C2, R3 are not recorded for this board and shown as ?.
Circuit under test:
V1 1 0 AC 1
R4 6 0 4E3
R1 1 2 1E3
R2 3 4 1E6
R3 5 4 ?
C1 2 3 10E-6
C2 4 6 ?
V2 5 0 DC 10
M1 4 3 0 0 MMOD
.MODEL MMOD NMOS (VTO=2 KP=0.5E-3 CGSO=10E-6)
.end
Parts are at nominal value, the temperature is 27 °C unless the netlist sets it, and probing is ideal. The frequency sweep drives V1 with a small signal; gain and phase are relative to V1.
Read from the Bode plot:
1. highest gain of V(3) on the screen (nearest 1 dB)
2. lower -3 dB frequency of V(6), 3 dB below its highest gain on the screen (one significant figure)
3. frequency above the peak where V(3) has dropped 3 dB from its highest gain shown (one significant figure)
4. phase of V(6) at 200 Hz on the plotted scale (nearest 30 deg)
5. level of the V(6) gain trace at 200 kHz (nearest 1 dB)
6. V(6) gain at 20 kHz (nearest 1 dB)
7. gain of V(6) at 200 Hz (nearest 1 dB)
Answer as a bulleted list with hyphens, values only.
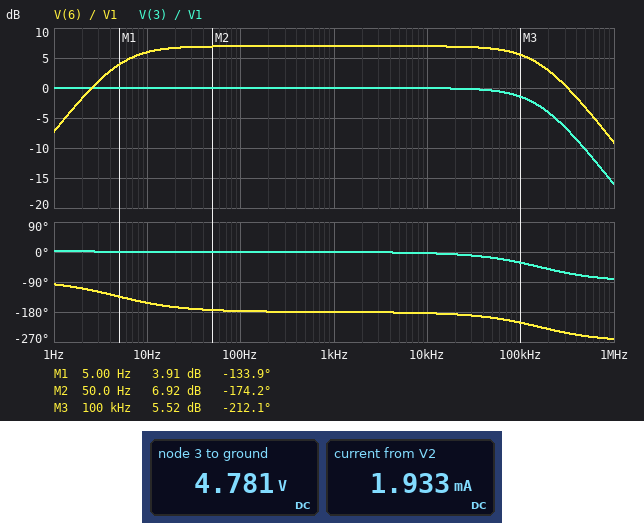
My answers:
- 0 dB
- 5 Hz
- 200 kHz
- -180 deg
- 3 dB
- 7 dB
- 7 dB
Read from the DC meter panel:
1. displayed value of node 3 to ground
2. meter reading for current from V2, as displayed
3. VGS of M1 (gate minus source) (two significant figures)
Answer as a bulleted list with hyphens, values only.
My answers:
- 4.781 V
- 1.933 mA
- 4.8 V
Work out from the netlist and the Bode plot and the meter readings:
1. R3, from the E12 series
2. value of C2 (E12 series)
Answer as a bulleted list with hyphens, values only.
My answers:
- 2.7 kΩ
- 4.7 µF
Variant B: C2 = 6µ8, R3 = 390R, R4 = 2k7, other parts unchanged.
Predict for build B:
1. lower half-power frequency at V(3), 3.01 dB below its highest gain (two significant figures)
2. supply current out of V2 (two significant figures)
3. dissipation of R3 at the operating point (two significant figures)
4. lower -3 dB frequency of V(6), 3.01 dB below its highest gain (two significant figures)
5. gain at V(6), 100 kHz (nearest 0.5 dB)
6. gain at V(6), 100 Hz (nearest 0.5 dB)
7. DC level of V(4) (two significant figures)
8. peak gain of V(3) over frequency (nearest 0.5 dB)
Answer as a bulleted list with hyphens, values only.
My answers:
- 32 mHz
- 7.0 mA
- 19 mW
- 7.6 Hz
- -2.5 dB
- -1.0 dB
- 7.3 V
- 0 dB
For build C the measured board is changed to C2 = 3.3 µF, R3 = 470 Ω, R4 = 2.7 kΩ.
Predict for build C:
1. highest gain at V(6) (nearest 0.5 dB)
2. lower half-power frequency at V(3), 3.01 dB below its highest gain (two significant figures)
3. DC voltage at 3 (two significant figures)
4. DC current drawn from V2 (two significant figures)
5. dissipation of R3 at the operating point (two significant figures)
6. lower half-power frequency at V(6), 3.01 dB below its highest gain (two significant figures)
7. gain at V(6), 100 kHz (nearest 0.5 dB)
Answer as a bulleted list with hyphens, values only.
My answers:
- 0 dB
- 35 mHz
- 7.0 V
- 6.3 mA
- 19 mW
- 15 Hz
- -1.5 dB
